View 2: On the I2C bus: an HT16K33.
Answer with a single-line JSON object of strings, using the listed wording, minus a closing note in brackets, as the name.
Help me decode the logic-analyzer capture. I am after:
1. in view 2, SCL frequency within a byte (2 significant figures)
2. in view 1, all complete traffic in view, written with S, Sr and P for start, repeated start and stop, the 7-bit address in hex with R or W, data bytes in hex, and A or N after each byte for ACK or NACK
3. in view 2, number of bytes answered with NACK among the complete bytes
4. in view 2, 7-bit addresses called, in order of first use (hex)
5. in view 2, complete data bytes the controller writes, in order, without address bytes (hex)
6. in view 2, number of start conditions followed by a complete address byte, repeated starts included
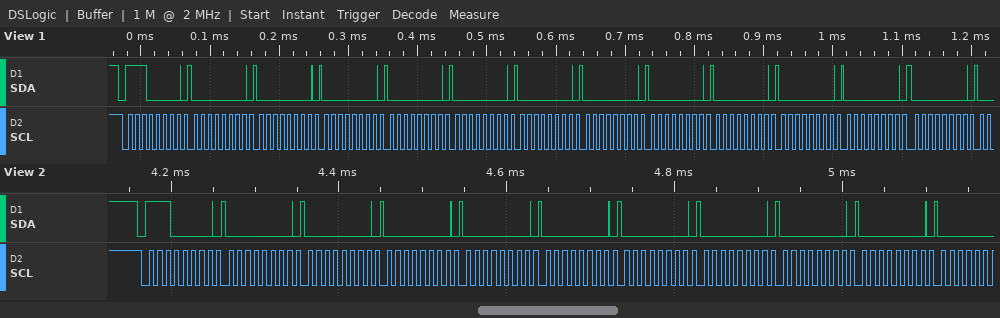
{"in view 2, SCL frequency within a byte": "100 kHz", "in view 1, all complete traffic in view, written with S, Sr and P for start, repeated start and stop, the 7-bit address in hex with R or W, data bytes in hex, and A or N after each byte for ACK or NACK": "S 70W A 00 A 00 A 00 A 00 A 00 A 00 A 00 A 00 A 00 A 00 A 00 A 00 A", "in view 2, number of bytes answered with NACK among the complete bytes": "0", "in view 2, 7-bit addresses called, in order of first use": "0x70", "in view 2, complete data bytes the controller writes, in order, without address bytes": "00 00 00 00 00 00 00 00 00", "in view 2, number of start conditions followed by a complete address byte, repeated starts included": "1"}
